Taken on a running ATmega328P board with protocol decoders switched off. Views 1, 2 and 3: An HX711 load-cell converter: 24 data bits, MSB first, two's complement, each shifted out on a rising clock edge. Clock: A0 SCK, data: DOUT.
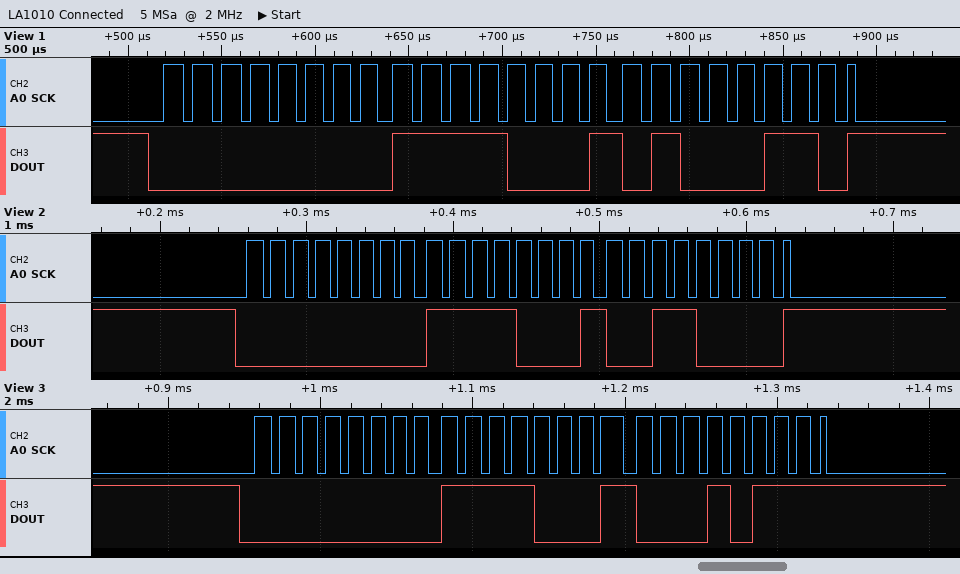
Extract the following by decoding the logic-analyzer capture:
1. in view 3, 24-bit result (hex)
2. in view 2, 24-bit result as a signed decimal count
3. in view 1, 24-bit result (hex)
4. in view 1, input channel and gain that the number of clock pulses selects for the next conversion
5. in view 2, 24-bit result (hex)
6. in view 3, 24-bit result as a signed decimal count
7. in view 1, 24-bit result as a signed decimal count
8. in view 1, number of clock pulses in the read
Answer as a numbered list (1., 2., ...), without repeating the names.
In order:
1. 0x00F117
2. 61744
3. 0x00F146
4. channel A, gain 128
5. 0x00F130
6. 61719
7. 61766
8. 25
